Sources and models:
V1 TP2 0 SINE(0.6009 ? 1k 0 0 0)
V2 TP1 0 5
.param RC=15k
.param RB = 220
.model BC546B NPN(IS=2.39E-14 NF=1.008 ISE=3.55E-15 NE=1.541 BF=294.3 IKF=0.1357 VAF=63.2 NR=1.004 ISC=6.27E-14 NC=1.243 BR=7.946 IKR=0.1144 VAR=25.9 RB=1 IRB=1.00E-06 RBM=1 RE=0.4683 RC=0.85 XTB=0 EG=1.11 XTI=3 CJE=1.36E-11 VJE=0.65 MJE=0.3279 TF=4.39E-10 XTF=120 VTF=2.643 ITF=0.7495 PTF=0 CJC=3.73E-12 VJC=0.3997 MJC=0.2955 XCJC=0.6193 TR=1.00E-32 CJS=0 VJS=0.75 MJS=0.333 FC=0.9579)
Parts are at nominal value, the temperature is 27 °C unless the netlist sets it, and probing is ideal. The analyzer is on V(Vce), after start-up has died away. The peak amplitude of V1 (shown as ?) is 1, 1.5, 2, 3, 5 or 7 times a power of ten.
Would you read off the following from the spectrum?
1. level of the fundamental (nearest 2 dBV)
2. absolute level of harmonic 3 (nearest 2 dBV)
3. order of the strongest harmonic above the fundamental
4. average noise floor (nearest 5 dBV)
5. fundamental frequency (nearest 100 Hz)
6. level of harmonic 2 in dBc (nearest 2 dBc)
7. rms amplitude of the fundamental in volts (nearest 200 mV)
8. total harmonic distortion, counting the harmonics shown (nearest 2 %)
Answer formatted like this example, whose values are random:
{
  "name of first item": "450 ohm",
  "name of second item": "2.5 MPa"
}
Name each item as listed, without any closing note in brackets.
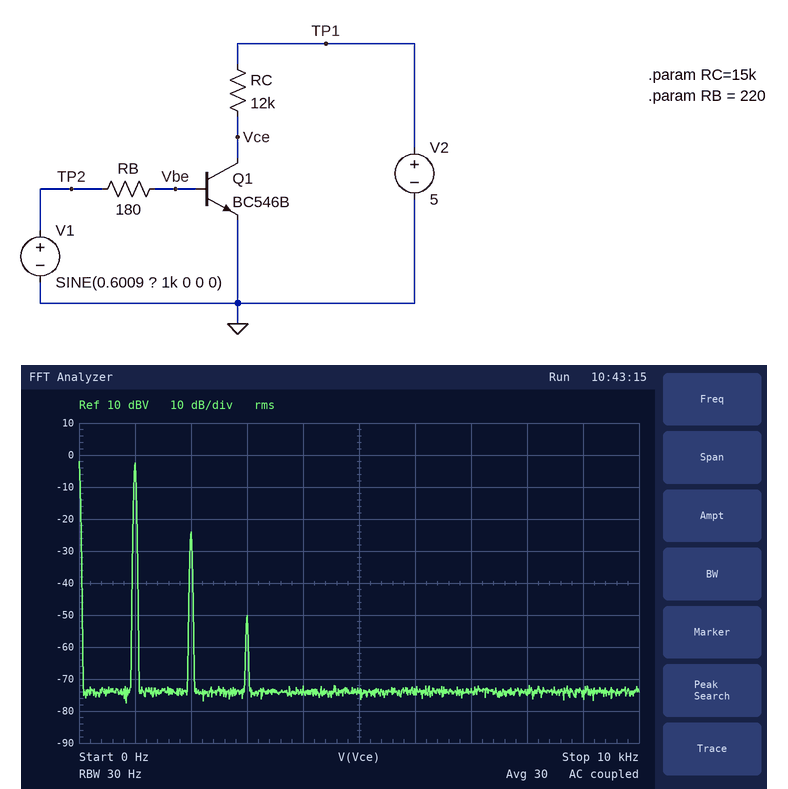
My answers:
{
  "level of the fundamental": "-2 dBV",
  "absolute level of harmonic 3": "-50 dBV",
  "order of the strongest harmonic above the fundamental": "2",
  "average noise floor": "-75 dBV",
  "fundamental frequency": "1.0 kHz",
  "level of harmonic 2 in dBc": "-22 dBc",
  "rms amplitude of the fundamental in volts": "800 mV",
  "total harmonic distortion, counting the harmonics shown": "8 %"
}
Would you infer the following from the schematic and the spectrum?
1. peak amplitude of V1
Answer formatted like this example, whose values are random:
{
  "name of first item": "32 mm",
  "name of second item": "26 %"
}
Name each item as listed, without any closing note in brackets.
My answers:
{
  "peak amplitude of V1": "10 mV"
}
